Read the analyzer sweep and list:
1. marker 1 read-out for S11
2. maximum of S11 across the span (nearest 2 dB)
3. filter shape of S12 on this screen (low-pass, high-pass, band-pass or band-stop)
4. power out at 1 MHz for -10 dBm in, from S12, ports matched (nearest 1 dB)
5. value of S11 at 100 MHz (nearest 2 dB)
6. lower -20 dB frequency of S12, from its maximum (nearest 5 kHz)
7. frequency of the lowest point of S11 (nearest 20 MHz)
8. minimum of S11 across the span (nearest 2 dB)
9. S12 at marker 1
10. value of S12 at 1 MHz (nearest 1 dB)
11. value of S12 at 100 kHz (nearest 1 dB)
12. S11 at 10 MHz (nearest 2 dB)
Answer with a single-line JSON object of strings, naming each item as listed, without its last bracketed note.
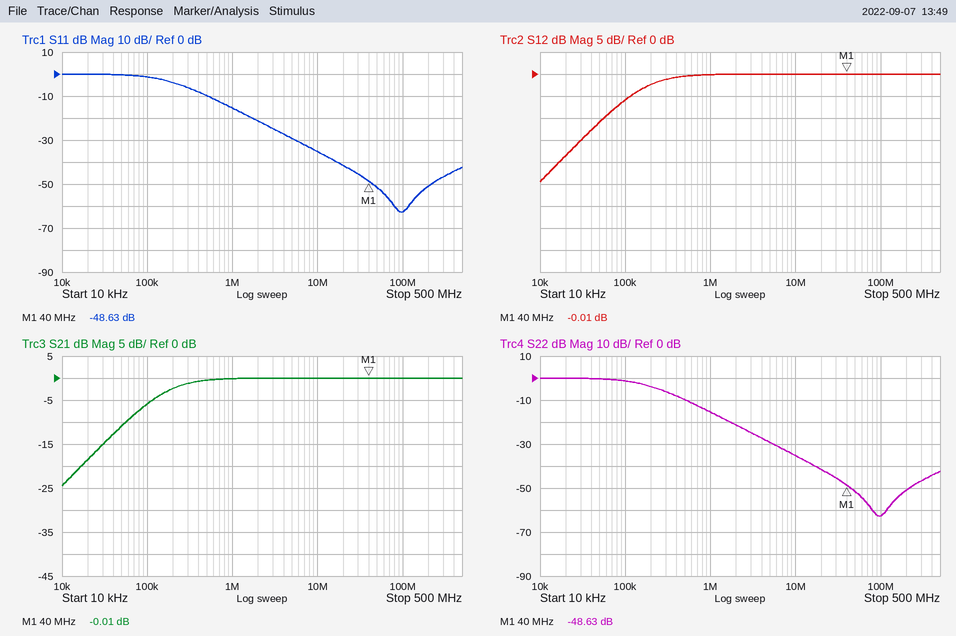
{"marker 1 read-out for S11": "-48.63 dB", "maximum of S11 across the span": "0 dB", "filter shape of S12 on this screen": "high-pass", "power out at 1 MHz for -10 dBm in, from S12, ports matched": "-10 dBm", "value of S11 at 100 MHz": "-62 dB", "lower -20 dB frequency of S12, from its maximum": "15 kHz", "frequency of the lowest point of S11": "100 MHz", "minimum of S11 across the span": "-62 dB", "S12 at marker 1": "-0.01 dB", "value of S12 at 1 MHz": "0 dB", "value of S12 at 100 kHz": "-6 dB", "S11 at 10 MHz": "-36 dB"}
